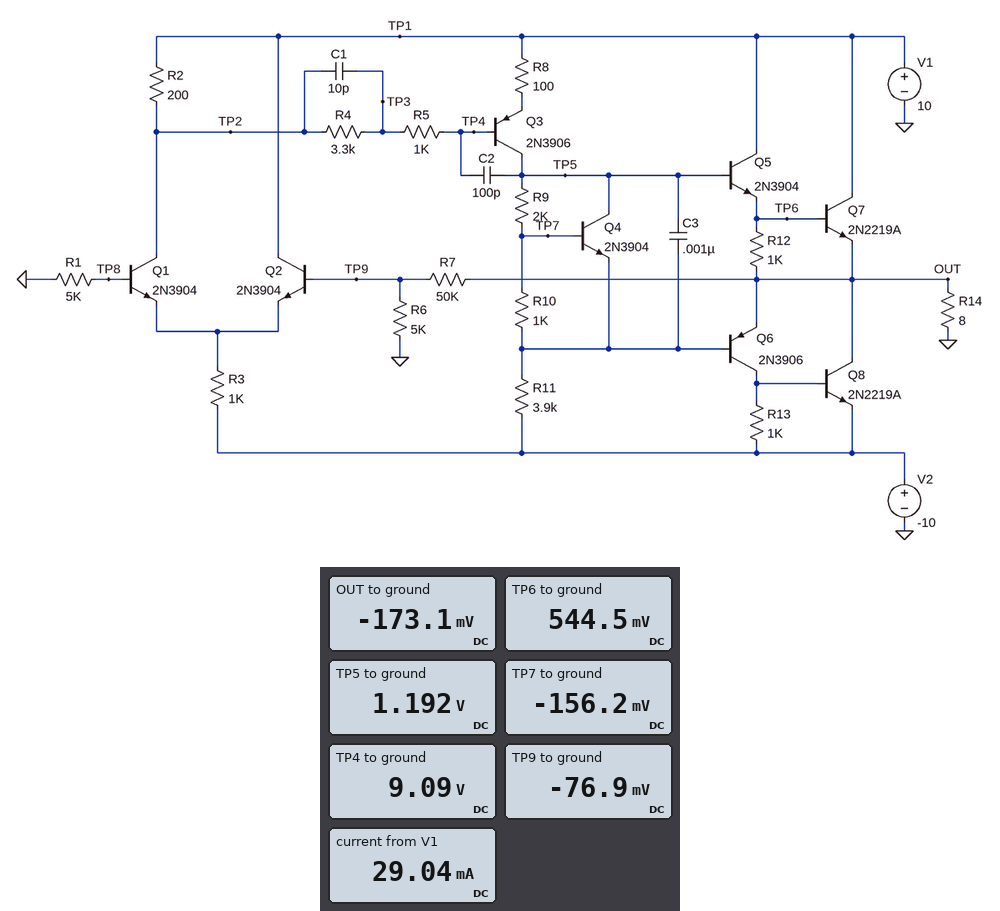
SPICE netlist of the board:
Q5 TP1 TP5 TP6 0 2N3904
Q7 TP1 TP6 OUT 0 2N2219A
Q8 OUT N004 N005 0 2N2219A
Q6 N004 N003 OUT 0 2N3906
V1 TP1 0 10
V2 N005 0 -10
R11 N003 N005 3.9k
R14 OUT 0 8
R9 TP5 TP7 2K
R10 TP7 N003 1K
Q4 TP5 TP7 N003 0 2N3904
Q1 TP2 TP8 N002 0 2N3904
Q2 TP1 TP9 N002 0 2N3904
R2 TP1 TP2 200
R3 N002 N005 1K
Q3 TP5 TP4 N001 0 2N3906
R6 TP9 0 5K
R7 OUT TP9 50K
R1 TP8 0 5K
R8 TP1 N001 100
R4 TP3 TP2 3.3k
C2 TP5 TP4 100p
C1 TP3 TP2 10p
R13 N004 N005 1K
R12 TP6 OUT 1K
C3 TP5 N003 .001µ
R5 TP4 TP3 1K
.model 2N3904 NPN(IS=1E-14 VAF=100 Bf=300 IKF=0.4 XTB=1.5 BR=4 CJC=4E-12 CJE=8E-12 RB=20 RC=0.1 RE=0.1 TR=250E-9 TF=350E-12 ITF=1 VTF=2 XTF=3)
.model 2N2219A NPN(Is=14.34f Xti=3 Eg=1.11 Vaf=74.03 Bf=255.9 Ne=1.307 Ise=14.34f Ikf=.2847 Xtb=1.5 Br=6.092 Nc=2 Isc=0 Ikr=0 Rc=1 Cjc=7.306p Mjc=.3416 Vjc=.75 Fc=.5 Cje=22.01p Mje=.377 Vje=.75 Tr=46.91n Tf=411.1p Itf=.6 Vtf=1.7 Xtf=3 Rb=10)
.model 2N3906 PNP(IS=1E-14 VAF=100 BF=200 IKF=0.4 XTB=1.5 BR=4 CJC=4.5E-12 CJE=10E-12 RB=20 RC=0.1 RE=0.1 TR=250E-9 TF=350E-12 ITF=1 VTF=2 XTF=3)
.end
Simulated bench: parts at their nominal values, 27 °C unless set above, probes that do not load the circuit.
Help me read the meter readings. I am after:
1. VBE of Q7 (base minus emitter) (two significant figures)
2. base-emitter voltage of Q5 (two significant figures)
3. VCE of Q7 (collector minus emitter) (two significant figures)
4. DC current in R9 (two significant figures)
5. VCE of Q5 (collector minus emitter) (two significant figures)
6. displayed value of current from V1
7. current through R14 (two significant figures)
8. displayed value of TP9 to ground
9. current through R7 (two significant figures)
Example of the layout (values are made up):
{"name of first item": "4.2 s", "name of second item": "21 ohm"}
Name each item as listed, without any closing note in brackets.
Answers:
{"VBE of Q7 (base minus emitter)": "720 mV", "base-emitter voltage of Q5": "650 mV", "VCE of Q7 (collector minus emitter)": "10 V", "DC current in R9": "670 µA", "VCE of Q5 (collector minus emitter)": "9.5 V", "displayed value of current from V1": "29.04 mA", "current through R14": "22 mA", "displayed value of TP9 to ground": "-76.9 mV", "current through R7": "1.9 µA"}
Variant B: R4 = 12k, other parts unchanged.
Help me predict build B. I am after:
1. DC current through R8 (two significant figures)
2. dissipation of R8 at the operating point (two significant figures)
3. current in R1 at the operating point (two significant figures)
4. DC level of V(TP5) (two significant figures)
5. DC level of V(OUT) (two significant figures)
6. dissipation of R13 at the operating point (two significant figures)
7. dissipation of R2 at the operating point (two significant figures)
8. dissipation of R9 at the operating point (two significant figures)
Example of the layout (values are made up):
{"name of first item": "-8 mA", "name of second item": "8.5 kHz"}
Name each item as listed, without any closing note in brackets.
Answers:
{"DC current through R8": "2.3 mA", "dissipation of R8 at the operating point": "530 µW", "current in R1 at the operating point": "16 µA", "DC level of V(TP5)": "990 mV", "DC level of V(OUT)": "-370 mV", "dissipation of R13 at the operating point": "570 µW", "dissipation of R2 at the operating point": "5.5 mW", "dissipation of R9 at the operating point": "910 µW"}
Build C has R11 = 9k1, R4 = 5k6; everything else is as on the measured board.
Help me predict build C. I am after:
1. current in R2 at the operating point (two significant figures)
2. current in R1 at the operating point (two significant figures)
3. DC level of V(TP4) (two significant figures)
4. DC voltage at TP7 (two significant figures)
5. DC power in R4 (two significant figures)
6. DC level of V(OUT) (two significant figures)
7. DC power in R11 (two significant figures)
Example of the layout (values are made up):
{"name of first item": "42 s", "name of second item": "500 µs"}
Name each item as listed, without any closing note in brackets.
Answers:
{"current in R2 at the operating point": "4.0 mA", "current in R1 at the operating point": "12 µA", "DC level of V(TP4)": "9.2 V", "DC voltage at TP7": "320 mV", "DC power in R4": "140 nW", "DC level of V(OUT)": "210 mV", "DC power in R11": "10 mW"}
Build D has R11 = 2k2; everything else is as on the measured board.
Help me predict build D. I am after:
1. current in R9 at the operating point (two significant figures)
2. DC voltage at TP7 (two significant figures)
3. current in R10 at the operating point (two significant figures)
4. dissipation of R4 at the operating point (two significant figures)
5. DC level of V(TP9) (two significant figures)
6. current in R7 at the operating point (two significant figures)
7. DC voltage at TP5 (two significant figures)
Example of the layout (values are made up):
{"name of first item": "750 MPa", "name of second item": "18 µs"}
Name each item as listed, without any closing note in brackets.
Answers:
{"current in R9 at the operating point": "700 µA", "DC voltage at TP7": "-640 mV", "current in R10 at the operating point": "690 µA", "dissipation of R4 at the operating point": "1.1 µW", "DC level of V(TP9)": "-110 mV", "current in R7 at the operating point": "11 µA", "DC voltage at TP5": "760 mV"}
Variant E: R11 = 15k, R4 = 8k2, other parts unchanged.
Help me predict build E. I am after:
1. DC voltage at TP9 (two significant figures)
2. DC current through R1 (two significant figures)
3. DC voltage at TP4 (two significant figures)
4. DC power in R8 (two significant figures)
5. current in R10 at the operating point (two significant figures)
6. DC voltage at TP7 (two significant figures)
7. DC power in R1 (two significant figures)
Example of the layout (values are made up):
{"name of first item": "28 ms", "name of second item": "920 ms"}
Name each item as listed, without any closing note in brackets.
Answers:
{"DC voltage at TP9": "-46 mV", "DC current through R1": "11 µA", "DC voltage at TP4": "9.3 V", "DC power in R8": "45 µW", "current in R10 at the operating point": "590 µA", "DC voltage at TP7": "560 mV", "DC power in R1": "650 nW"}
